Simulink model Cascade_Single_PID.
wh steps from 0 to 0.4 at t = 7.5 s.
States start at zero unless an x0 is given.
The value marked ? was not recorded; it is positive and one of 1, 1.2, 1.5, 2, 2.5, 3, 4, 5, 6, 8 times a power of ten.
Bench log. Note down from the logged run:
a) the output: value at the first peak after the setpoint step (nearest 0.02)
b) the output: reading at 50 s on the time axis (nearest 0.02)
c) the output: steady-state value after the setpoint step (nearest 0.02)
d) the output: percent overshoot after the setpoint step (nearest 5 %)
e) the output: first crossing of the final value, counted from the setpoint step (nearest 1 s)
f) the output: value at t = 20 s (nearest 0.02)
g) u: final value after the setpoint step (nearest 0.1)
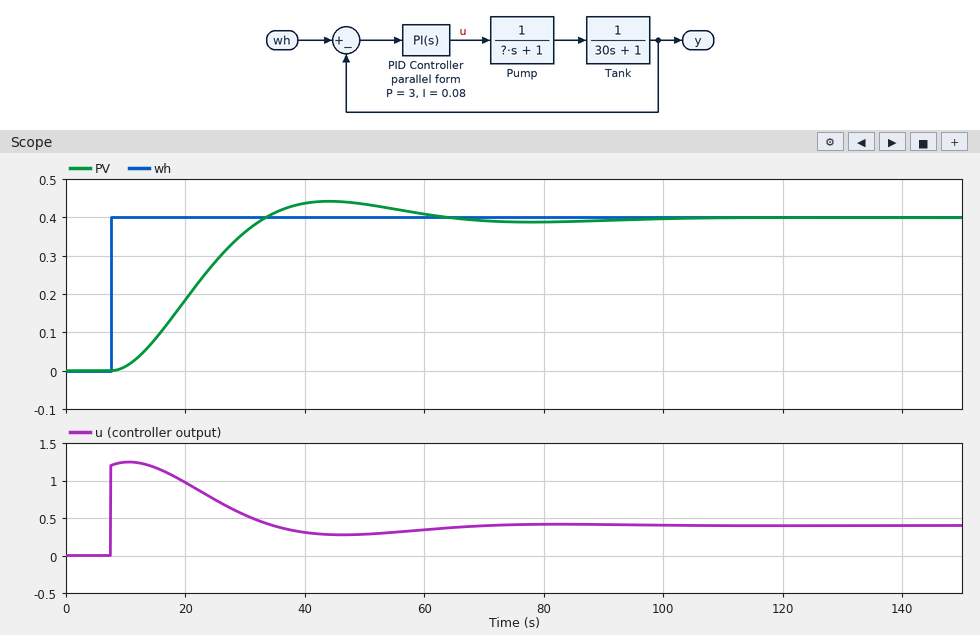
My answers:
0.44
0.44
0.40
10 %
26 s
0.18
0.4
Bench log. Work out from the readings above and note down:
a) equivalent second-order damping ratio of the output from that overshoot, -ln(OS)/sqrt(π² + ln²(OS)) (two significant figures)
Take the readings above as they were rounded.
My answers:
0.59
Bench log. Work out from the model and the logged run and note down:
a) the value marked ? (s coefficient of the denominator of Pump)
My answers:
10
